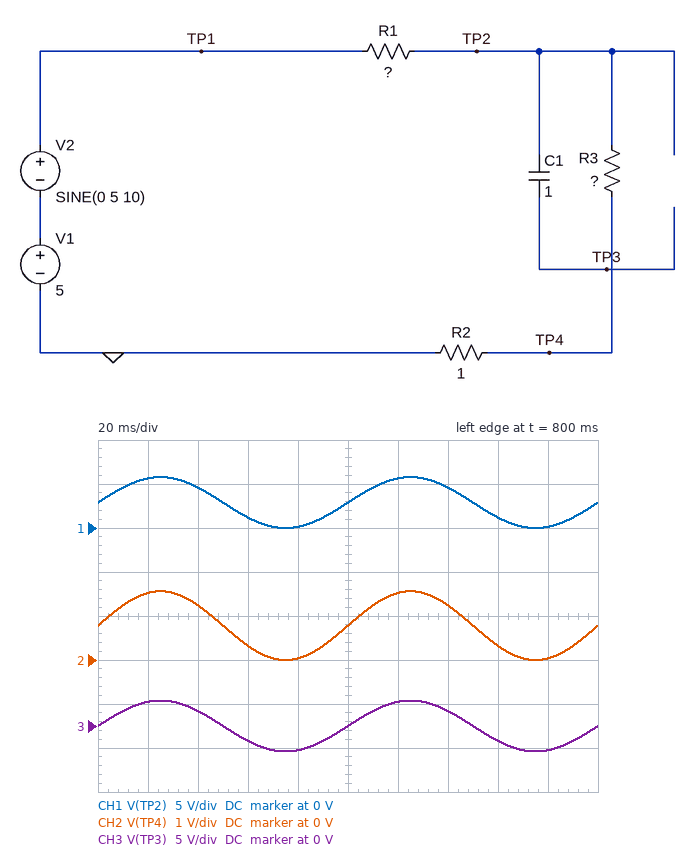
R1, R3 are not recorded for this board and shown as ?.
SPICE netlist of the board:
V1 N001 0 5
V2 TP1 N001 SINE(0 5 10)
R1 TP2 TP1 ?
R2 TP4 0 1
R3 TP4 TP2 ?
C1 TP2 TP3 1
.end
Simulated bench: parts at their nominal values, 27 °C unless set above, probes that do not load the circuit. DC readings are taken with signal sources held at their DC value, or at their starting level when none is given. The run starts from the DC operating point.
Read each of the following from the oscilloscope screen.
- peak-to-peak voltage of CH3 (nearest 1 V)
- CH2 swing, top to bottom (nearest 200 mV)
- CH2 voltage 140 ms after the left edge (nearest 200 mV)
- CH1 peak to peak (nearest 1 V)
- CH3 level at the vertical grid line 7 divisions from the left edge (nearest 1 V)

6 V
1.6 V
1.2 V
6 V
2 V
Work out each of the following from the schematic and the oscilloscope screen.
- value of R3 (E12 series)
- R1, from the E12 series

2.7 Ω
2.7 Ω
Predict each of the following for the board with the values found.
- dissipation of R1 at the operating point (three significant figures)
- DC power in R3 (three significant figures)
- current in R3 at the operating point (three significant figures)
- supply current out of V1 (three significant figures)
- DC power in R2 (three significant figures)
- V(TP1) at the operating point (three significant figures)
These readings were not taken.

1.65 W
1.65 W
781 mA
781 mA
610 mW
5.00 V
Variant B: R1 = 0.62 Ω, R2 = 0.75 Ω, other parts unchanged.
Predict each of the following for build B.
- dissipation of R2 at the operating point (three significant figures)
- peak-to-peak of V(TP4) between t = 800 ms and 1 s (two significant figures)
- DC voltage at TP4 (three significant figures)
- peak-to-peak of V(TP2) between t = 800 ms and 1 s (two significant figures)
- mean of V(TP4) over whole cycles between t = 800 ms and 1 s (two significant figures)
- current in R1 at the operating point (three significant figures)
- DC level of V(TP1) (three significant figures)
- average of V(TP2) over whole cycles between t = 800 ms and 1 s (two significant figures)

1.13 W
1.8 V
921 mV
8.5 V
920 mV
1.23 A
5.00 V
4.2 V
